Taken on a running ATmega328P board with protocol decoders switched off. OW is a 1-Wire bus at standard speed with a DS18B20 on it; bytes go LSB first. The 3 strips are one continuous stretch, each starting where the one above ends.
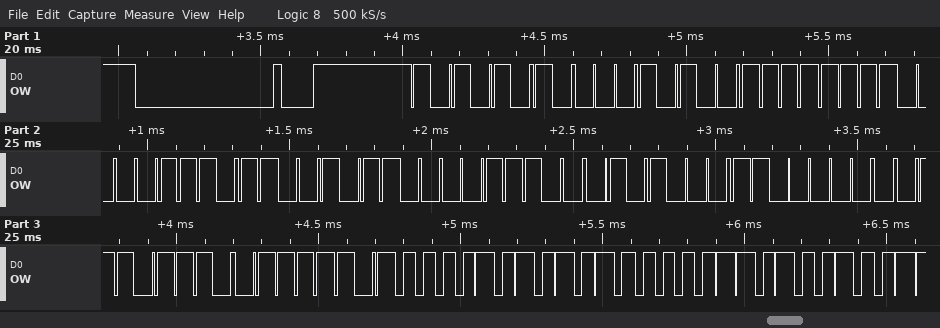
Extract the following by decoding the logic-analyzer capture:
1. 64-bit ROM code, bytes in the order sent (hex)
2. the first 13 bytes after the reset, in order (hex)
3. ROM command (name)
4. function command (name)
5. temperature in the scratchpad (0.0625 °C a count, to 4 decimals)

28 FF 70 D3 70 14 03 76
55 28 FF 70 D3 70 14 03 76 BE 50 05 4B
Match ROM
Read Scratchpad
85.0000 °C
